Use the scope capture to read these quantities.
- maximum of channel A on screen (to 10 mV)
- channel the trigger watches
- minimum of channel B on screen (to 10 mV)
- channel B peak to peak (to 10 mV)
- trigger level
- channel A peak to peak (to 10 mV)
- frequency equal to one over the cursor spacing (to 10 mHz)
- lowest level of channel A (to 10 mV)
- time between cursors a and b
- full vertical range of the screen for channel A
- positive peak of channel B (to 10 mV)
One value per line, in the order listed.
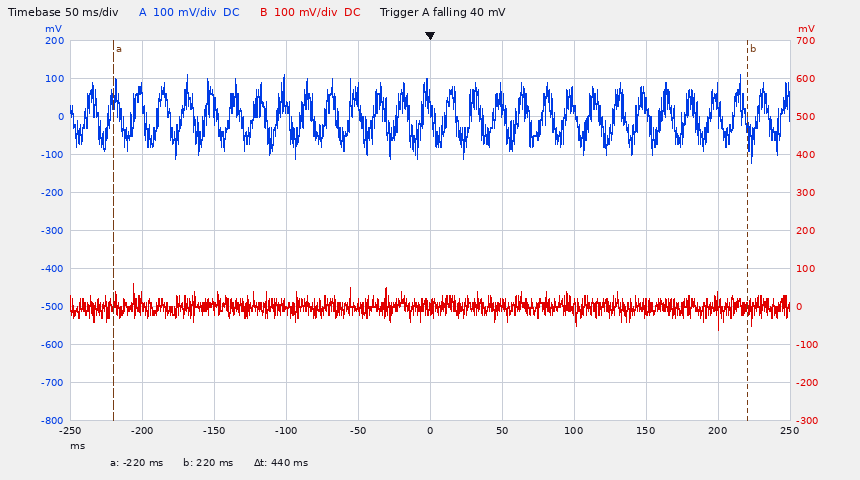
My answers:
110 mV
channel A
-60 mV
120 mV
40 mV
230 mV
2.27 Hz
-120 mV
440 ms
1 V
60 mV
